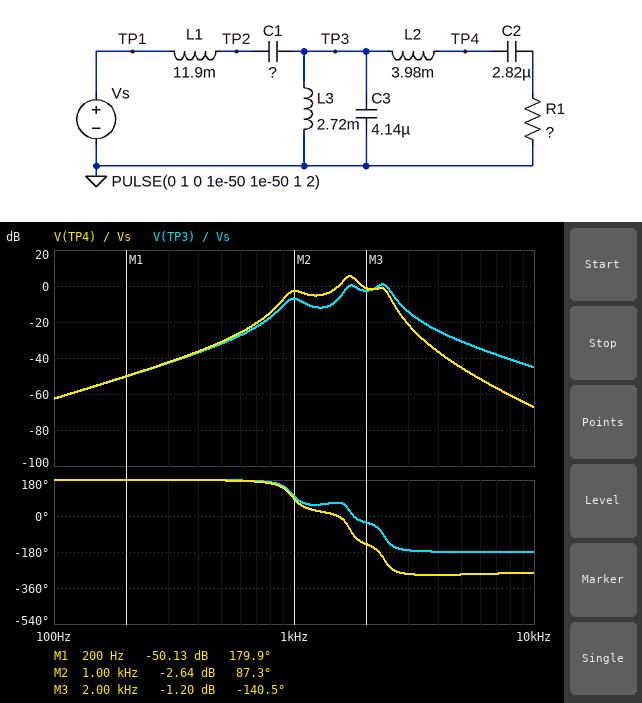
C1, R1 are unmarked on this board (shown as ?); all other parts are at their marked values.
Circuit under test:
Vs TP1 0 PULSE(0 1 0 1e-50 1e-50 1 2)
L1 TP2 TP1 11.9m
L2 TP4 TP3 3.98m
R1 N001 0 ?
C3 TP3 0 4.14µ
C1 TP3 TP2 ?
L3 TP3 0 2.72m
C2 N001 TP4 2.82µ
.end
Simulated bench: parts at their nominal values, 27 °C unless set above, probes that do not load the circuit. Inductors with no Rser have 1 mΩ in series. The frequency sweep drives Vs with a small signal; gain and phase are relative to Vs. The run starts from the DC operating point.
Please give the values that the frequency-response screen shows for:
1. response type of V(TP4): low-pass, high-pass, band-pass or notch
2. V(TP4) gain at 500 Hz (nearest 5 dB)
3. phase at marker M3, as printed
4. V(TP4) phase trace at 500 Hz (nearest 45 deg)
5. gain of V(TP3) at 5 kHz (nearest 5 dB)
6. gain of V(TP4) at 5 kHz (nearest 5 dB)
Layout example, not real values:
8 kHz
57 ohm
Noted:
band-pass
-30 dB
-140.5 deg
180 deg
-30 dB
-45 dB
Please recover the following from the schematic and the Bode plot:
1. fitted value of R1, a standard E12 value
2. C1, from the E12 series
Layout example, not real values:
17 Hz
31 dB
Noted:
18 Ω
680 nF
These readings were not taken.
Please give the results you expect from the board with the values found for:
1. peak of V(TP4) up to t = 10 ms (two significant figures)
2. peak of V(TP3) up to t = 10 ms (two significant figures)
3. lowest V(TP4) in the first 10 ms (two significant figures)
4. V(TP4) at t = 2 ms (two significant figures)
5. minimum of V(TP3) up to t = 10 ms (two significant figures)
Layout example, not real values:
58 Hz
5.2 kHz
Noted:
240 mV
130 mV
-300 mV
110 mV
-220 mV
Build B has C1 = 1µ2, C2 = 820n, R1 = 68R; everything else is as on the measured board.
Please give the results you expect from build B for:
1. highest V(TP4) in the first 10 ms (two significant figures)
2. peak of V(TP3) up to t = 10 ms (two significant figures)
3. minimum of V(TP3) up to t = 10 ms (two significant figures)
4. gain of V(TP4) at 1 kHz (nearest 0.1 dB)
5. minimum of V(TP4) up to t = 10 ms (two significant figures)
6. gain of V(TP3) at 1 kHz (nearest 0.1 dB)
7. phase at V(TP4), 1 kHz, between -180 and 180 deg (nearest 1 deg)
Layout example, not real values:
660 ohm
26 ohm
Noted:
450 mV
360 mV
-370 mV
5.5 dB
-460 mV
4.5 dB
166 deg
